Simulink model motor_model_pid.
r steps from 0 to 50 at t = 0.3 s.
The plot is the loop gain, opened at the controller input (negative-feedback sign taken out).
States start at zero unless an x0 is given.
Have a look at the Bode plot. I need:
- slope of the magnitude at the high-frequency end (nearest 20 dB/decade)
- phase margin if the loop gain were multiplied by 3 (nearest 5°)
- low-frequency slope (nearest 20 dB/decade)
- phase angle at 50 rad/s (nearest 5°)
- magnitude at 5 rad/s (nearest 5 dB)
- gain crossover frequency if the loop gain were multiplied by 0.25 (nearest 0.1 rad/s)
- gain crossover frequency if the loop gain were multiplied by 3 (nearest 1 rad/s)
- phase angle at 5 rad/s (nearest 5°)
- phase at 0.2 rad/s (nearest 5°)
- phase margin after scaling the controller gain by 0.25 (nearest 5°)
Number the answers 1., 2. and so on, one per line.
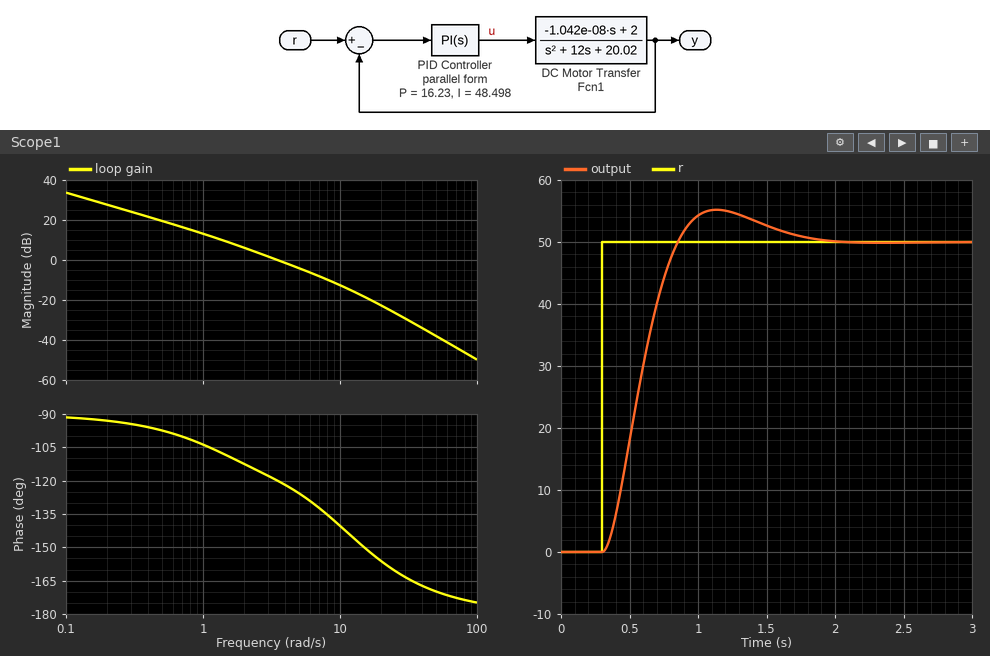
1. -40 dB/decade
2. 45°
3. -20 dB/decade
4. -170°
5. -5 dB
6. 1.1 rad/s
7. 8 rad/s
8. -125°
9. -95°
10. 75°
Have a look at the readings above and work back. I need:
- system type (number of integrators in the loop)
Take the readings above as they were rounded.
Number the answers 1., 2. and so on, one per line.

1. 1
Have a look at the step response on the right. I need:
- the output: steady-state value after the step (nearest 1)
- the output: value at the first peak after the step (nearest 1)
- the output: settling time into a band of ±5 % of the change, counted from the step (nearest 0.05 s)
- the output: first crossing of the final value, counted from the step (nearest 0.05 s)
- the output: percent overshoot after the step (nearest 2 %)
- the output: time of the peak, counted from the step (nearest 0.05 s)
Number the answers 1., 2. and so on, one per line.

1. 50
2. 55
3. 1.20 s
4. 0.55 s
5. 10 %
6. 0.85 s
